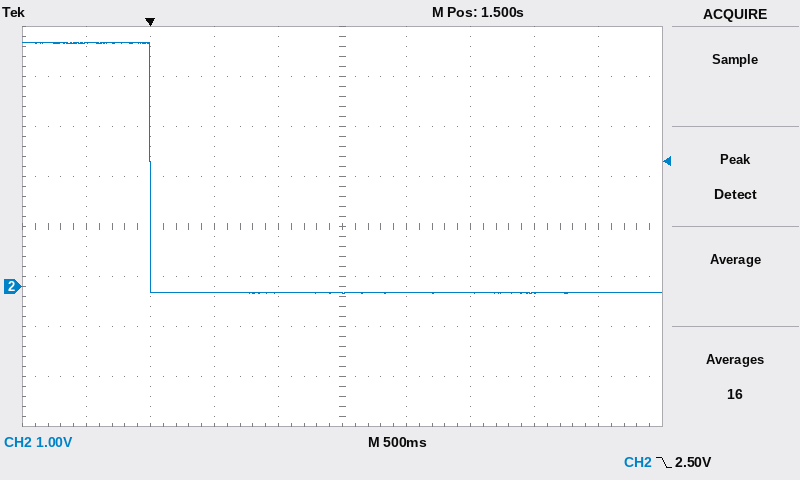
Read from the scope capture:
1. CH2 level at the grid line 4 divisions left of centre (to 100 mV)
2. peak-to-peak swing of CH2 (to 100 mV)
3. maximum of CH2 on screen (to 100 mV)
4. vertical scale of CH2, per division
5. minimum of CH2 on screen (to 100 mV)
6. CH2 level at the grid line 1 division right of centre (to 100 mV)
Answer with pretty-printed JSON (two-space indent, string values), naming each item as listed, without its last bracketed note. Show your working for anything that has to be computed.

{
  "CH2 level at the grid line 4 divisions left of centre": "4.9 V",
  "peak-to-peak swing of CH2": "4.9 V − (-100 mV) = 5.0 V",
  "maximum of CH2 on screen": "4.9 V",
  "vertical scale of CH2, per division": "1 V",
  "minimum of CH2 on screen": "-100 mV",
  "CH2 level at the grid line 1 division right of centre": "-100 mV"
}
